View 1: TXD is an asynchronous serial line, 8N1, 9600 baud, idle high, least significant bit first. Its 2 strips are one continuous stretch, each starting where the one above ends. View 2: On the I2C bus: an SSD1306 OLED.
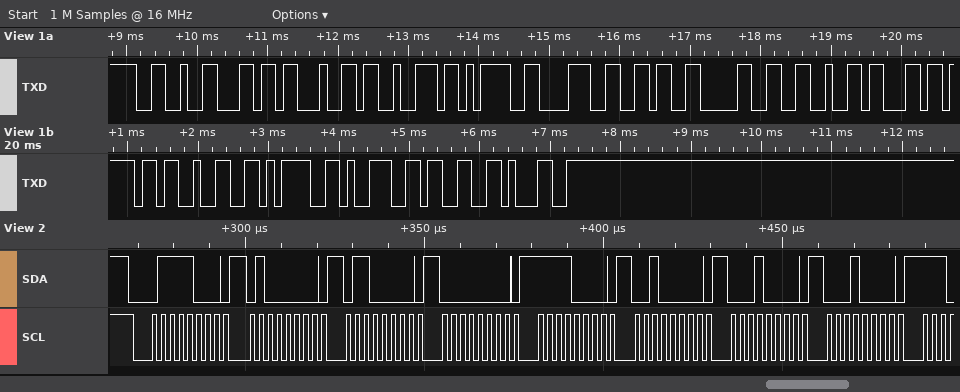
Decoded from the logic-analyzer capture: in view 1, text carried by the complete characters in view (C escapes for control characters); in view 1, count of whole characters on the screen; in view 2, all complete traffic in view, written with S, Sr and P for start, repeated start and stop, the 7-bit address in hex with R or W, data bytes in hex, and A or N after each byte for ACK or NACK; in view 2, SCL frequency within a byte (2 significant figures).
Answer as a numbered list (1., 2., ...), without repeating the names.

1. "&ldr=860&co2=931"
2. 16
3. S 3CW A 40 A 60 A 00 A F0 A 20 A 10 A 10 A
4. 400 kHz
